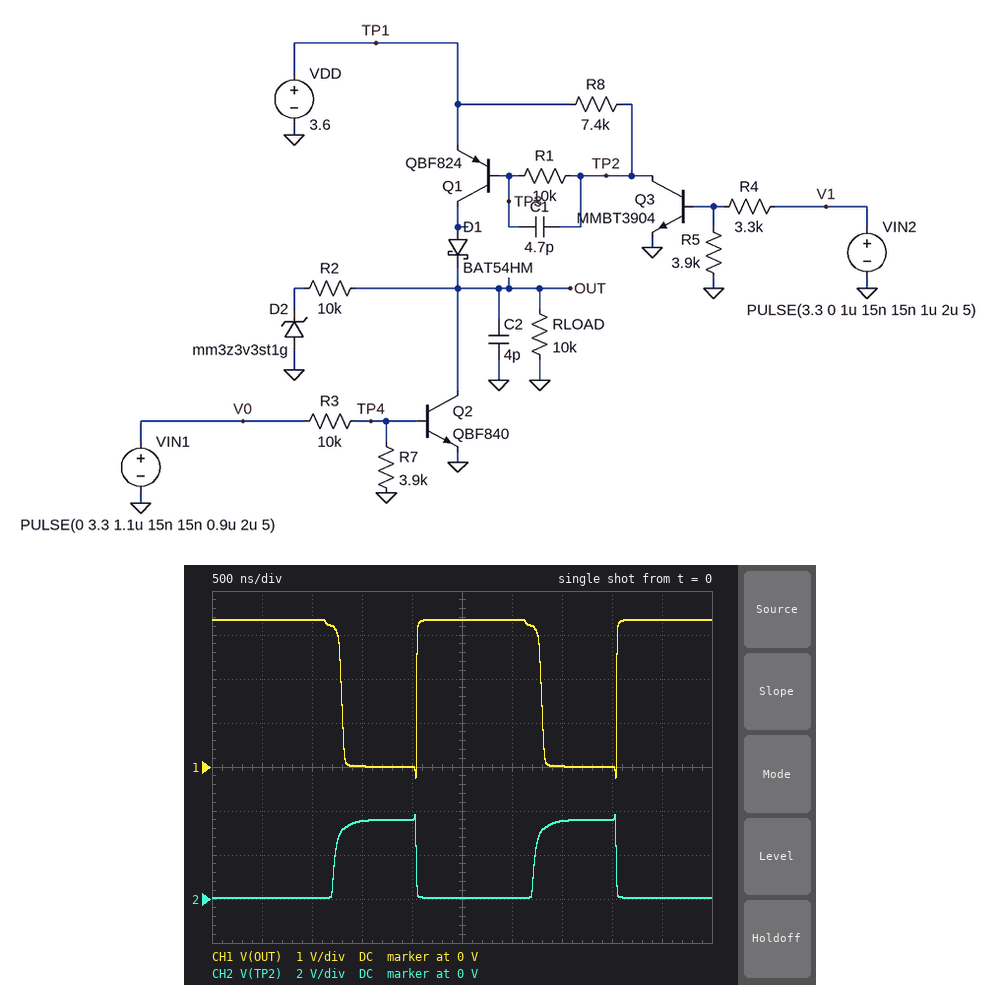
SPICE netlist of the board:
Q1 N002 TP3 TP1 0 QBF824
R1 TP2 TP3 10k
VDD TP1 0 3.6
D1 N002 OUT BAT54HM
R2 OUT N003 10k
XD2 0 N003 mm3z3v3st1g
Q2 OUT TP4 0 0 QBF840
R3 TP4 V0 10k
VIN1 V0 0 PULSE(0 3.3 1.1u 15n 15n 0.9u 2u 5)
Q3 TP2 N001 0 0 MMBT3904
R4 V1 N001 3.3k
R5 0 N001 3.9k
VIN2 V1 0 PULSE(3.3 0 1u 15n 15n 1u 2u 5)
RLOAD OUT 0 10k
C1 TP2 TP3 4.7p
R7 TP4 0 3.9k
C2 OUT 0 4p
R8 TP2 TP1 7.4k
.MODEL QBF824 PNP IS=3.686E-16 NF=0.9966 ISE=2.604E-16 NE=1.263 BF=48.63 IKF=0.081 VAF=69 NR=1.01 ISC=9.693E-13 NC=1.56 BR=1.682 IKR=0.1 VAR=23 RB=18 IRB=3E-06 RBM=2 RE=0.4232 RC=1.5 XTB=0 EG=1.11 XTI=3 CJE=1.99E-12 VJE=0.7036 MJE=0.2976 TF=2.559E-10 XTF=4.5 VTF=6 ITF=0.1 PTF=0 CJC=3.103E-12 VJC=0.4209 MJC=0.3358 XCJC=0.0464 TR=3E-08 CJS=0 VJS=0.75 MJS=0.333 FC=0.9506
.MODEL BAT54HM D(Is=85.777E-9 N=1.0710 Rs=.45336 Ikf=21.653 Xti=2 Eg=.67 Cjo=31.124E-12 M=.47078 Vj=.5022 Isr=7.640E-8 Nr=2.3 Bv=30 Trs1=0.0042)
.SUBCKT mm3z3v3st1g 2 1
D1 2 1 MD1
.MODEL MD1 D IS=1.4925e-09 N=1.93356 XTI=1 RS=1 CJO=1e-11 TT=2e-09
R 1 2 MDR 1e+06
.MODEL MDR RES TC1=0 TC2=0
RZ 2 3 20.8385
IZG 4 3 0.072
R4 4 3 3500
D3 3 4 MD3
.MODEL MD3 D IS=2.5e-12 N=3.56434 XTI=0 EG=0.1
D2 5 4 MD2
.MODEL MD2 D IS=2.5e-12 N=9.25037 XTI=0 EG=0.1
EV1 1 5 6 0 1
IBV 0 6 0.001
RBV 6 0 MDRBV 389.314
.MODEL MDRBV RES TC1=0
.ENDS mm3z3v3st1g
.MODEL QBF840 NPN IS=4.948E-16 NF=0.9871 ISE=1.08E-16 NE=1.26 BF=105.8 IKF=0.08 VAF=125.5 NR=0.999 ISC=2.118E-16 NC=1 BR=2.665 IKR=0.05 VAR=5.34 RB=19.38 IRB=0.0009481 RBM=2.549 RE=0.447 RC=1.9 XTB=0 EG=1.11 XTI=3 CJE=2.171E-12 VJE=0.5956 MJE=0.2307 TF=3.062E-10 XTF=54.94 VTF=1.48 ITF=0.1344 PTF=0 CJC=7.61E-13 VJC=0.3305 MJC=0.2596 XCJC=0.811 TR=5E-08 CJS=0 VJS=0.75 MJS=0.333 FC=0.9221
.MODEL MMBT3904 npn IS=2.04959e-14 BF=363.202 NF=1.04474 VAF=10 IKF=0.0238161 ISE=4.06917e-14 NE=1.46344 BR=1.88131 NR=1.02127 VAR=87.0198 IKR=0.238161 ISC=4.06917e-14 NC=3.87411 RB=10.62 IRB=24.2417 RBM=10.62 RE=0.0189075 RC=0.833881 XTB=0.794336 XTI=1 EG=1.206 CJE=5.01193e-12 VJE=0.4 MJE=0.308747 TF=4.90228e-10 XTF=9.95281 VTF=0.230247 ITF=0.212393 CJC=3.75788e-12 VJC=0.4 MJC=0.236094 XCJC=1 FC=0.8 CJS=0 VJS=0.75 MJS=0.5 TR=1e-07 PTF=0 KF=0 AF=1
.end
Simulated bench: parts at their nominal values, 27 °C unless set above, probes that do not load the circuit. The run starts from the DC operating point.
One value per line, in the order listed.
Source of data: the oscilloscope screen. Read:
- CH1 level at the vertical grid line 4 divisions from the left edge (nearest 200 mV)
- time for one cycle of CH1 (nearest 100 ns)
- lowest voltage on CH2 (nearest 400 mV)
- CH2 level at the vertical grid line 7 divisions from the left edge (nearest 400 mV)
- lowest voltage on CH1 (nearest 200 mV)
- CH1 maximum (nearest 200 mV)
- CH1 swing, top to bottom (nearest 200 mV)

0 V
2.0 µs
0 V
3.6 V
-200 mV
3.4 V
3.6 V
